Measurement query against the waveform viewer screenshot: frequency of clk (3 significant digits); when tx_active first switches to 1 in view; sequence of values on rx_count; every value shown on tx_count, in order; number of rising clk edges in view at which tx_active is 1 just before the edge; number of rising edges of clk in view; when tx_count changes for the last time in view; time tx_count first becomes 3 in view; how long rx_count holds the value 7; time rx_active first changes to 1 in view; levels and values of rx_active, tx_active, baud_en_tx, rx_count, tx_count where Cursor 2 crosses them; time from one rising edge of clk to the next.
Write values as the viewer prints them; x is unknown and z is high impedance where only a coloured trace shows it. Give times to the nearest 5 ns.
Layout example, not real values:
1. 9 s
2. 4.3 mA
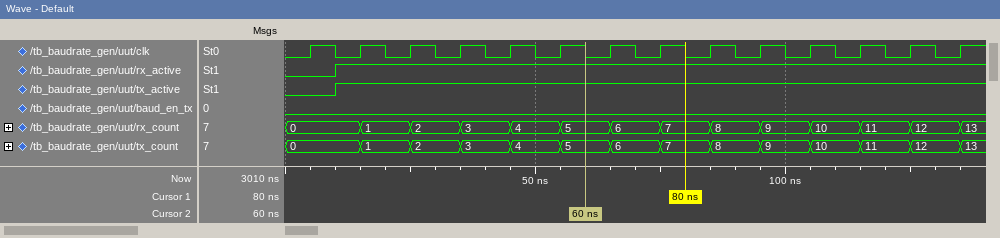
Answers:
1. 100 MHz
2. 10 ns
3. 0, 1, 2, 3, 4, 5, 6, 7, 8, 9, 10, 11, 12, 13
4. 0, 1, 2, 3, 4, 5, 6, 7, 8, 9, 10, 11, 12, 13
5. 13
6. 14
7. 135 ns
8. 35 ns
9. 10 ns
10. 10 ns
11. rx_active=1, tx_active=1, baud_en_tx=0, rx_count=5, tx_count=5
12. 10 ns
